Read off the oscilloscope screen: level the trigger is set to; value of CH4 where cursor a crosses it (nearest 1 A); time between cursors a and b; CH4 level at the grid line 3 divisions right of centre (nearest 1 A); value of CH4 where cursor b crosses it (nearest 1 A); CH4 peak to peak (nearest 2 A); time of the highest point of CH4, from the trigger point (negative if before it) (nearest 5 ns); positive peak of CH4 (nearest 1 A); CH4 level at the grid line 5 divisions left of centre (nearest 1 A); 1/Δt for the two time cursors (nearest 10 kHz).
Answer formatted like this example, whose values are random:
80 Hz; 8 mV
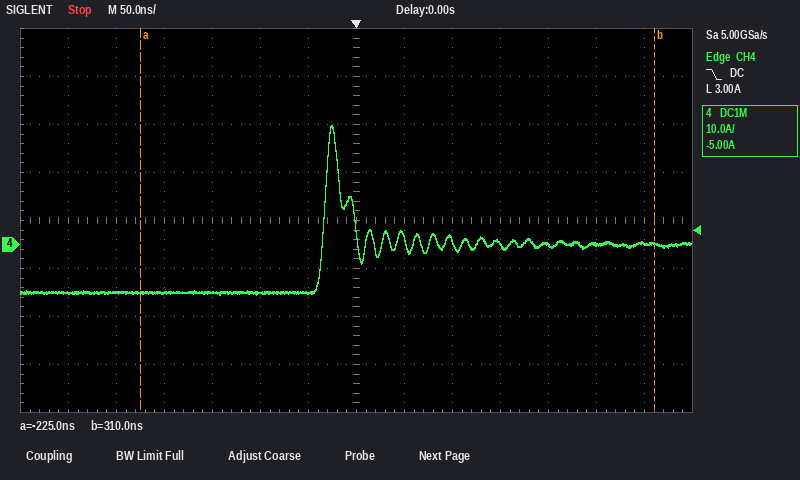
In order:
3.00 A; -10 A; 535 ns; 0 A; 0 A; 36 A; -25 ns; 25 A; -10 A; 1.87 MHz
